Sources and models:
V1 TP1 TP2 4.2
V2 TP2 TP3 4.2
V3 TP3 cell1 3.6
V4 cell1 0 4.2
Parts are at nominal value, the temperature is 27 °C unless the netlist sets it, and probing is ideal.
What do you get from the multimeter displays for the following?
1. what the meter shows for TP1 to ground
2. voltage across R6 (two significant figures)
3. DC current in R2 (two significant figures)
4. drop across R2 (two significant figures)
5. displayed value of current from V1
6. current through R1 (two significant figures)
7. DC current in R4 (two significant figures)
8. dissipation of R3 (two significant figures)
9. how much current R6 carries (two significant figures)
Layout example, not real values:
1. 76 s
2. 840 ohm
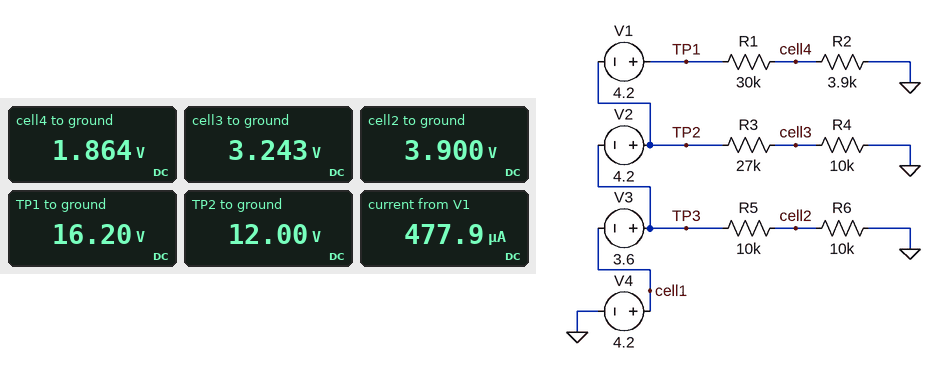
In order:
1. 16.20 V
2. 3.9 V
3. 480 µA
4. 1.9 V
5. 477.9 µA
6. 480 µA
7. 320 µA
8. 2.8 mW
9. 390 µA
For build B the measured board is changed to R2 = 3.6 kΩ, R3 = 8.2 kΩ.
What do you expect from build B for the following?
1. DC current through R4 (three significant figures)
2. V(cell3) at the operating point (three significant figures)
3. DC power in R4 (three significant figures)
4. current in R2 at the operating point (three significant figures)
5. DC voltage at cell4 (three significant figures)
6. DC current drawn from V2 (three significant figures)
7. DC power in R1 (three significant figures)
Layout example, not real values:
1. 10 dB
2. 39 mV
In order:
1. 659 µA
2. 6.59 V
3. 4.35 mW
4. 482 µA
5. 1.74 V
6. 1.14 mA
7. 6.97 mW
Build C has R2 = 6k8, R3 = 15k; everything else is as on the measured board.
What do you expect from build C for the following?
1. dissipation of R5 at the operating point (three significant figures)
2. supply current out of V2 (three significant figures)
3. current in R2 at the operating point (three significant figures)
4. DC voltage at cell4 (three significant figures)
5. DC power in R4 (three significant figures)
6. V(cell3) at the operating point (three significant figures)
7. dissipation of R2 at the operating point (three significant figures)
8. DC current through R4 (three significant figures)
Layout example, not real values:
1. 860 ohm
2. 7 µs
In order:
1. 1.52 mW
2. 920 µA
3. 440 µA
4. 2.99 V
5. 2.30 mW
6. 4.80 V
7. 1.32 mW
8. 480 µA
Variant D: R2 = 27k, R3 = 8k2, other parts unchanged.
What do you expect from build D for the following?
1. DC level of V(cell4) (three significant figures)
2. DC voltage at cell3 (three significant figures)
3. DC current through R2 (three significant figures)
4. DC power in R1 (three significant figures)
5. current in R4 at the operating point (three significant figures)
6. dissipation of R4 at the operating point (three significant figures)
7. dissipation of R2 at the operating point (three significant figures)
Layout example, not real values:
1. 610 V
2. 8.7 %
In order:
1. 7.67 V
2. 6.59 V
3. 284 µA
4. 2.42 mW
5. 659 µA
6. 4.35 mW
7. 2.18 mW
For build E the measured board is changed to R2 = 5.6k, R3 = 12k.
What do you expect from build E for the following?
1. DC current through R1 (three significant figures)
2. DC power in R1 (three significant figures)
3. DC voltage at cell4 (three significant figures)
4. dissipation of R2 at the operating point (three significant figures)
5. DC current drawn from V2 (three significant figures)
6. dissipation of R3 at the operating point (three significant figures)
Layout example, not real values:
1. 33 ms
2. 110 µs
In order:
1. 455 µA
2. 6.21 mW
3. 2.55 V
4. 1.16 mW
5. 1.00 mA
6. 3.57 mW
